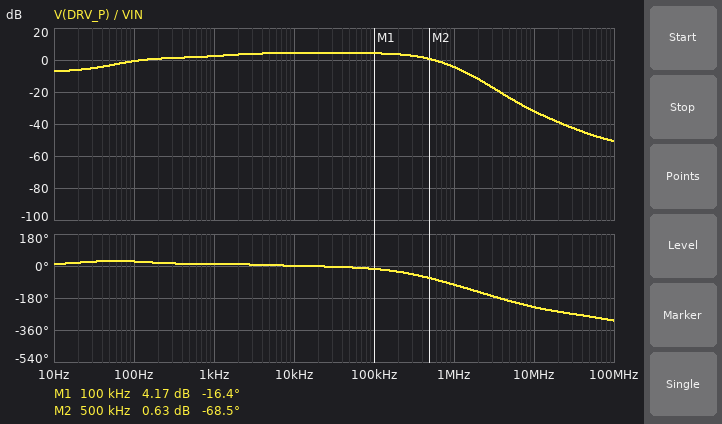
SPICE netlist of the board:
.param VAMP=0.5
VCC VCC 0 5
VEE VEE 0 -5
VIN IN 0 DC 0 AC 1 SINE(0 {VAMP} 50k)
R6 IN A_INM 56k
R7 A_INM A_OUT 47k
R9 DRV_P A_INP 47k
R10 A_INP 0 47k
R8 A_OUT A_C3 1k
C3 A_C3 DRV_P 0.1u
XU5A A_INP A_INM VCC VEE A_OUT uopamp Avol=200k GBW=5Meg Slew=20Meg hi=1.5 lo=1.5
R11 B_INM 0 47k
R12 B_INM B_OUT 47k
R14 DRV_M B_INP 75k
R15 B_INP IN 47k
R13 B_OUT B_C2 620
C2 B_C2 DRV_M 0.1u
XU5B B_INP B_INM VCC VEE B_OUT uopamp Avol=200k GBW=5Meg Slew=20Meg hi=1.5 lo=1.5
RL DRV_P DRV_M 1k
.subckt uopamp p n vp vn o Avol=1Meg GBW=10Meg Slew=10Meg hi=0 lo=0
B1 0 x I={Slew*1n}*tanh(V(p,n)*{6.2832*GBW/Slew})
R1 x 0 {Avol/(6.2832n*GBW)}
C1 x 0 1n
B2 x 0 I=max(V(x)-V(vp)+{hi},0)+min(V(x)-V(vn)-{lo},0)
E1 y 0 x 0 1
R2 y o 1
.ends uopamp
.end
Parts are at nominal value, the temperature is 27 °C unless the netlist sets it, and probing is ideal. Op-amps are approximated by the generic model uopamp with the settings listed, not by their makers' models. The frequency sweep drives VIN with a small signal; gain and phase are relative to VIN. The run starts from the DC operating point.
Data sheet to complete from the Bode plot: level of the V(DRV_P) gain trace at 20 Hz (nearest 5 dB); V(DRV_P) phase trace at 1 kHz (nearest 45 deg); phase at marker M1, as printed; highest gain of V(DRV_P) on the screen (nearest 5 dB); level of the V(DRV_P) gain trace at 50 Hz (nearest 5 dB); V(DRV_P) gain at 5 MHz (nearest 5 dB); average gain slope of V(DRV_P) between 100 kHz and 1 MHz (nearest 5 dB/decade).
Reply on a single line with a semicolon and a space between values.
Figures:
-5 dB; 0 deg; -16.4 deg; 5 dB; -5 dB; -25 dB; -10 dB/decade
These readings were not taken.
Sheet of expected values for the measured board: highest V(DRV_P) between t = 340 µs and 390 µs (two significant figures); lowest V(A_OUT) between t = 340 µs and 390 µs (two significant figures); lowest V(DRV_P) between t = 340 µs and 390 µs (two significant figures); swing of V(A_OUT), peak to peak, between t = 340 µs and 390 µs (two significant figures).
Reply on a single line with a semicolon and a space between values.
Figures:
820 mV; -350 mV; -820 mV; 690 mV
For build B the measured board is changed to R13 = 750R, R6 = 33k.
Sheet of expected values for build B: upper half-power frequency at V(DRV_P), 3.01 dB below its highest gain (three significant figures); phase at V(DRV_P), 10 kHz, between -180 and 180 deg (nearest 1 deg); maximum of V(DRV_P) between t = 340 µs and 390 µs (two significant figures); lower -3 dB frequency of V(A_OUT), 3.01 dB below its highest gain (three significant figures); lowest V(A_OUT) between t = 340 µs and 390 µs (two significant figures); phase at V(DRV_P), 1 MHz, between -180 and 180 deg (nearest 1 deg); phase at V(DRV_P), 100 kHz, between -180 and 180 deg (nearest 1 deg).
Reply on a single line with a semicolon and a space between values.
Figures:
38.4 kHz; 170 deg; 1.5 V; 634 Hz; -2.4 V; 127 deg; 124 deg
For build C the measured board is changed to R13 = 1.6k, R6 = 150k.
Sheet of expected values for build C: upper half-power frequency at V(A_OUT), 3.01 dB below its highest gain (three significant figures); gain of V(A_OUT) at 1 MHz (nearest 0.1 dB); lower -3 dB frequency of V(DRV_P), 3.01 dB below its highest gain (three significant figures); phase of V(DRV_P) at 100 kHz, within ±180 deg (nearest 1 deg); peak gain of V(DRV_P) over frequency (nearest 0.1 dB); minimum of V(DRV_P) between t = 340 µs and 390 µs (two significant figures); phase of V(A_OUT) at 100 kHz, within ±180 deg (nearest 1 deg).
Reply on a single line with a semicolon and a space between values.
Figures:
1.25 kHz; -9.4 dB; 42.6 Hz; -9 deg; 3.5 dB; -370 mV; -26 deg
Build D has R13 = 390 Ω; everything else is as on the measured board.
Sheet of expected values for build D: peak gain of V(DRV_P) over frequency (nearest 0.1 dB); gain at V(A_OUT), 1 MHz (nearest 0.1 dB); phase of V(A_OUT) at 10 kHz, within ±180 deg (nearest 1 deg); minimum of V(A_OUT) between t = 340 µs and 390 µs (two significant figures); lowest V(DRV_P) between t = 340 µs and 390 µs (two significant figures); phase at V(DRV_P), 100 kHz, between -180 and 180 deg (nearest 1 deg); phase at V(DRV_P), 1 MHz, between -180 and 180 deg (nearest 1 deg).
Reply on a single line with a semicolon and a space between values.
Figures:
7.8 dB; 1.4 dB; 6 deg; -710 mV; -1.2 V; -15 deg; -96 deg
